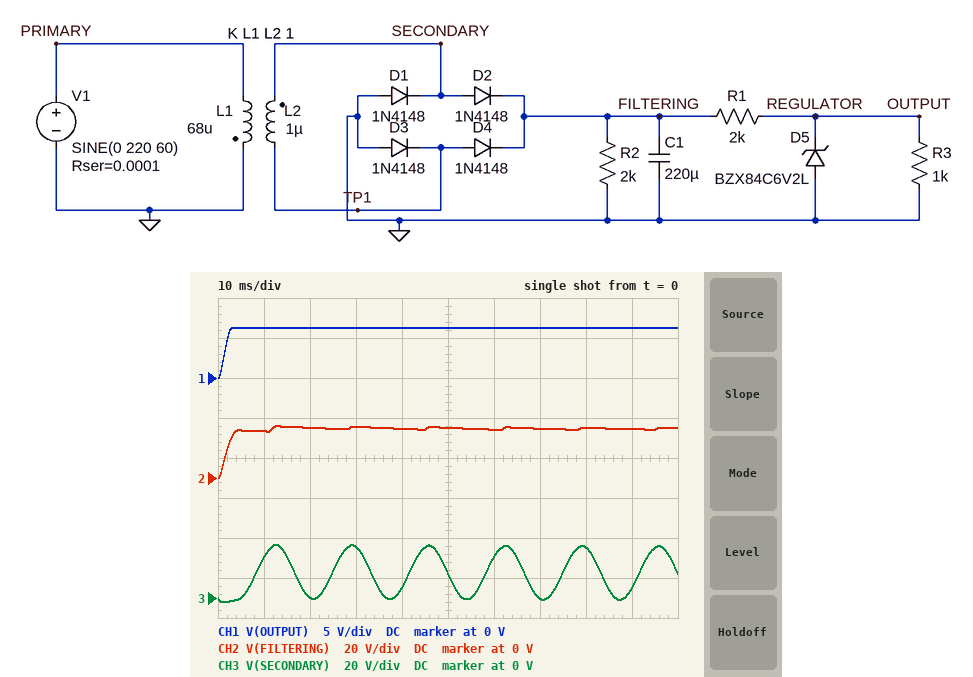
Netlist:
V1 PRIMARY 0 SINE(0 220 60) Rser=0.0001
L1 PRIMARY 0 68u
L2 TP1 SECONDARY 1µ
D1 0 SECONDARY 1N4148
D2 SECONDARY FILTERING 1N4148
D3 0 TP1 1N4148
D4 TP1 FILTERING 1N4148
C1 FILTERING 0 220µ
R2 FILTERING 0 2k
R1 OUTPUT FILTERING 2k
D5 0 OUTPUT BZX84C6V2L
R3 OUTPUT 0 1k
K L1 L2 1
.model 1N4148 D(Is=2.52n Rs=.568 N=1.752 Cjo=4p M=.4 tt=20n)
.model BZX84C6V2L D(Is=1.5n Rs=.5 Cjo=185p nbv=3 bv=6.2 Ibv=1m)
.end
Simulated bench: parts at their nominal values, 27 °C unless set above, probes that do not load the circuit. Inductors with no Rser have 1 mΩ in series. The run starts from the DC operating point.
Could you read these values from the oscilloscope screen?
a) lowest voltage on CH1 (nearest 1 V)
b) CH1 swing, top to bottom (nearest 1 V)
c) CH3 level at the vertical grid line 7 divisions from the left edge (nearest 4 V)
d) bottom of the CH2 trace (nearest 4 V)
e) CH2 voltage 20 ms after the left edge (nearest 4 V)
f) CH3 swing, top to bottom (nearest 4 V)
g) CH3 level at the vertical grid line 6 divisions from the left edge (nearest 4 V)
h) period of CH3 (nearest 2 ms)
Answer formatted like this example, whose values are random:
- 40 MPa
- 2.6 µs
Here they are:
- 0 V
- 6 V
- 0 V
- 0 V
- 24 V
- 28 V
- 20 V
- 16 ms
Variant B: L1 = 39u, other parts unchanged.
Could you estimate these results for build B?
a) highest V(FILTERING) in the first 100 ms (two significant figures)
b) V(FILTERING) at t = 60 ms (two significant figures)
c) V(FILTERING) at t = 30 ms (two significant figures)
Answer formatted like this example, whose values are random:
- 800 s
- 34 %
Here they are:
- 35 V
- 32 V
- 34 V
